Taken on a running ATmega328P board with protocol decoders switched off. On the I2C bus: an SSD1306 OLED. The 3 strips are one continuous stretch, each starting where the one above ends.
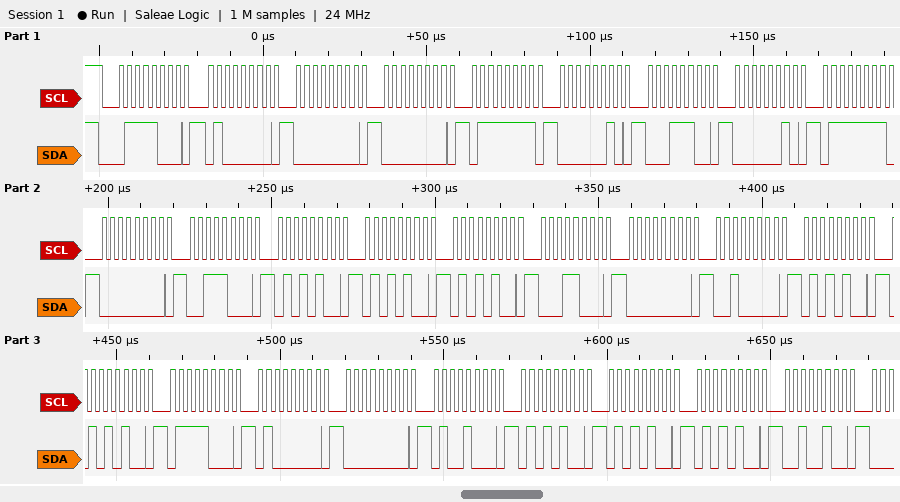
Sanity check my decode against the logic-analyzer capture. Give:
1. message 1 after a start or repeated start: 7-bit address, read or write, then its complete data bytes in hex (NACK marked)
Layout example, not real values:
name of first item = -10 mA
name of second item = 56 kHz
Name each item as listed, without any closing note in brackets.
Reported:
message 1 after a start or repeated start: 7-bit address, read or write, then its complete data bytes in hex = 0x3C write: 40 00 00 7F 02 1C 02 7F 00 38 54 54 54 18 00 20 54 54 78 40 00 48 54 54 54 24
